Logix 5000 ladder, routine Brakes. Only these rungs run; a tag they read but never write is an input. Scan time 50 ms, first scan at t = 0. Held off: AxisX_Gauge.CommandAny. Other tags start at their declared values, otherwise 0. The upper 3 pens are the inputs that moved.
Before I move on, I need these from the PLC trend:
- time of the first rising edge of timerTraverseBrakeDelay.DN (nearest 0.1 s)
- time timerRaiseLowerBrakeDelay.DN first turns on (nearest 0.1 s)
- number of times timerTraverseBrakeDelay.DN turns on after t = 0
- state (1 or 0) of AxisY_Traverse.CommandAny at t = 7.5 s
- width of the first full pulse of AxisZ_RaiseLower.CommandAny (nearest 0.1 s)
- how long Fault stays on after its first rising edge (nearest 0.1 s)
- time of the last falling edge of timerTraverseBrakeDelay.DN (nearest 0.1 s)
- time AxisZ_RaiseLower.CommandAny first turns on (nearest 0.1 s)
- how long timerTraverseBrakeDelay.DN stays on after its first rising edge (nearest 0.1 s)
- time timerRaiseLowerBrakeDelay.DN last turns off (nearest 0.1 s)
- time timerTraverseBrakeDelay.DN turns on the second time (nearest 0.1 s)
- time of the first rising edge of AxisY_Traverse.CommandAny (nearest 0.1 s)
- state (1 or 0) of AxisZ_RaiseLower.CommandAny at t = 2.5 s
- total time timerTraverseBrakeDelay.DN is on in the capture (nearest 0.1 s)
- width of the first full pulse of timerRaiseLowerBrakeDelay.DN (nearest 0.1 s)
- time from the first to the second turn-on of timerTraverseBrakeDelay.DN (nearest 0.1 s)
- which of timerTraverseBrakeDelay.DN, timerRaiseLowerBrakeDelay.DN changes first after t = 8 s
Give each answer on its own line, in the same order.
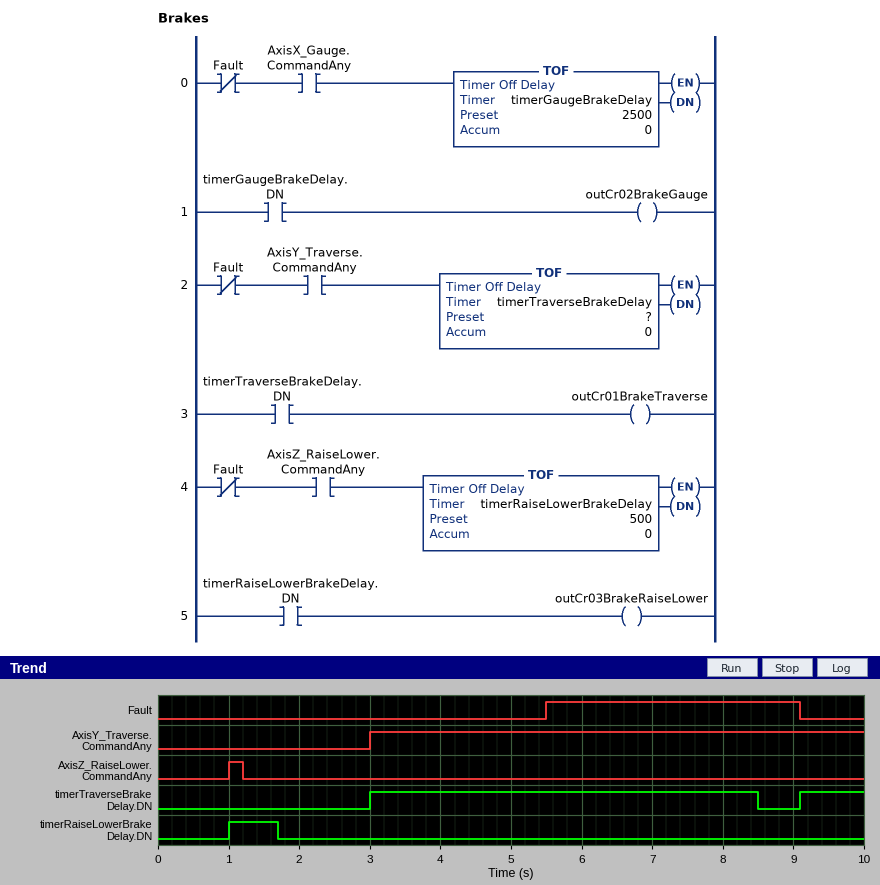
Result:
3.0 s
1.0 s
2
1
0.2 s
3.6 s
8.5 s
1.0 s
5.5 s
1.7 s
9.1 s
3.0 s
0
6.4 s
0.7 s
6.1 s
timerTraverseBrakeDelay.DN
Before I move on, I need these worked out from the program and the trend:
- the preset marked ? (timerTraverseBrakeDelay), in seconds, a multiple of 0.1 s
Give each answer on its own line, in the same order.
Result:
3.0 s
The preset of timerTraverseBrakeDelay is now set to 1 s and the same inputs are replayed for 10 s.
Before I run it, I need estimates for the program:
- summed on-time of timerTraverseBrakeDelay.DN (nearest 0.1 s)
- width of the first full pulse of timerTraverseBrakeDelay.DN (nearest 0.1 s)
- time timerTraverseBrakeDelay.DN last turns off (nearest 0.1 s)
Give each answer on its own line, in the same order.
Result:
4.4 s
3.5 s
6.5 s
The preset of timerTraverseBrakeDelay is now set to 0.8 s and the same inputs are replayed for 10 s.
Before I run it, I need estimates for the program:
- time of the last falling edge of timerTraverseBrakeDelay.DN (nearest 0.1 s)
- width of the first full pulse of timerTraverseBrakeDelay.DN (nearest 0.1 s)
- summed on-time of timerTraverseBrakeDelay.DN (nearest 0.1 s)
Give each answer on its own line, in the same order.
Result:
6.3 s
3.3 s
4.2 s
